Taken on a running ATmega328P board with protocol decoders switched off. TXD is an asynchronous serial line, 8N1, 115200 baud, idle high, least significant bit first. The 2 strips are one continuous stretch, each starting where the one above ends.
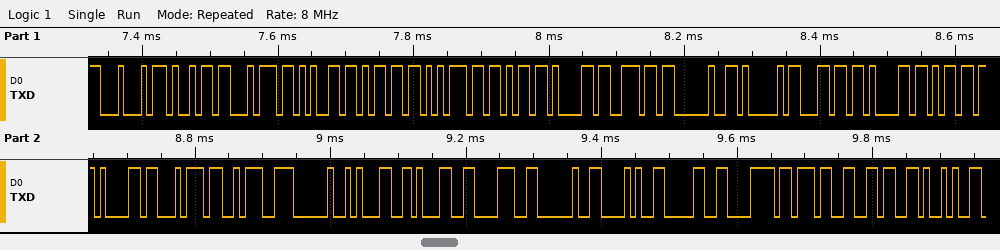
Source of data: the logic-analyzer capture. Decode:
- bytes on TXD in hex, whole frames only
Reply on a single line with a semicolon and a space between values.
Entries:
44 69 74 65 6D 75 6B 61 6E 20 41 6C 61 6D 61 74 3A 20 31 31 38 20 28 30 78 37 36 29
